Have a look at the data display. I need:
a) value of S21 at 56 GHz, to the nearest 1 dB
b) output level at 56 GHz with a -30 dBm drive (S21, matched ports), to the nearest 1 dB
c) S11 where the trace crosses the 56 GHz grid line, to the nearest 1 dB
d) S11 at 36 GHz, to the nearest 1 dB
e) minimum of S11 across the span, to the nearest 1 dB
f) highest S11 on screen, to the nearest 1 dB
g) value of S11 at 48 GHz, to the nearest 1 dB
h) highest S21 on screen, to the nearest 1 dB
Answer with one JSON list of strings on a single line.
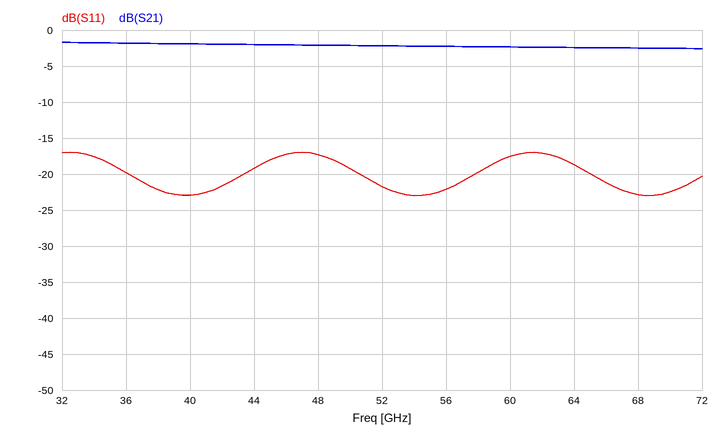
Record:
["-2 dB", "-32 dBm", "-22 dB", "-20 dB", "-23 dB", "-17 dB", "-17 dB", "-2 dB"]
